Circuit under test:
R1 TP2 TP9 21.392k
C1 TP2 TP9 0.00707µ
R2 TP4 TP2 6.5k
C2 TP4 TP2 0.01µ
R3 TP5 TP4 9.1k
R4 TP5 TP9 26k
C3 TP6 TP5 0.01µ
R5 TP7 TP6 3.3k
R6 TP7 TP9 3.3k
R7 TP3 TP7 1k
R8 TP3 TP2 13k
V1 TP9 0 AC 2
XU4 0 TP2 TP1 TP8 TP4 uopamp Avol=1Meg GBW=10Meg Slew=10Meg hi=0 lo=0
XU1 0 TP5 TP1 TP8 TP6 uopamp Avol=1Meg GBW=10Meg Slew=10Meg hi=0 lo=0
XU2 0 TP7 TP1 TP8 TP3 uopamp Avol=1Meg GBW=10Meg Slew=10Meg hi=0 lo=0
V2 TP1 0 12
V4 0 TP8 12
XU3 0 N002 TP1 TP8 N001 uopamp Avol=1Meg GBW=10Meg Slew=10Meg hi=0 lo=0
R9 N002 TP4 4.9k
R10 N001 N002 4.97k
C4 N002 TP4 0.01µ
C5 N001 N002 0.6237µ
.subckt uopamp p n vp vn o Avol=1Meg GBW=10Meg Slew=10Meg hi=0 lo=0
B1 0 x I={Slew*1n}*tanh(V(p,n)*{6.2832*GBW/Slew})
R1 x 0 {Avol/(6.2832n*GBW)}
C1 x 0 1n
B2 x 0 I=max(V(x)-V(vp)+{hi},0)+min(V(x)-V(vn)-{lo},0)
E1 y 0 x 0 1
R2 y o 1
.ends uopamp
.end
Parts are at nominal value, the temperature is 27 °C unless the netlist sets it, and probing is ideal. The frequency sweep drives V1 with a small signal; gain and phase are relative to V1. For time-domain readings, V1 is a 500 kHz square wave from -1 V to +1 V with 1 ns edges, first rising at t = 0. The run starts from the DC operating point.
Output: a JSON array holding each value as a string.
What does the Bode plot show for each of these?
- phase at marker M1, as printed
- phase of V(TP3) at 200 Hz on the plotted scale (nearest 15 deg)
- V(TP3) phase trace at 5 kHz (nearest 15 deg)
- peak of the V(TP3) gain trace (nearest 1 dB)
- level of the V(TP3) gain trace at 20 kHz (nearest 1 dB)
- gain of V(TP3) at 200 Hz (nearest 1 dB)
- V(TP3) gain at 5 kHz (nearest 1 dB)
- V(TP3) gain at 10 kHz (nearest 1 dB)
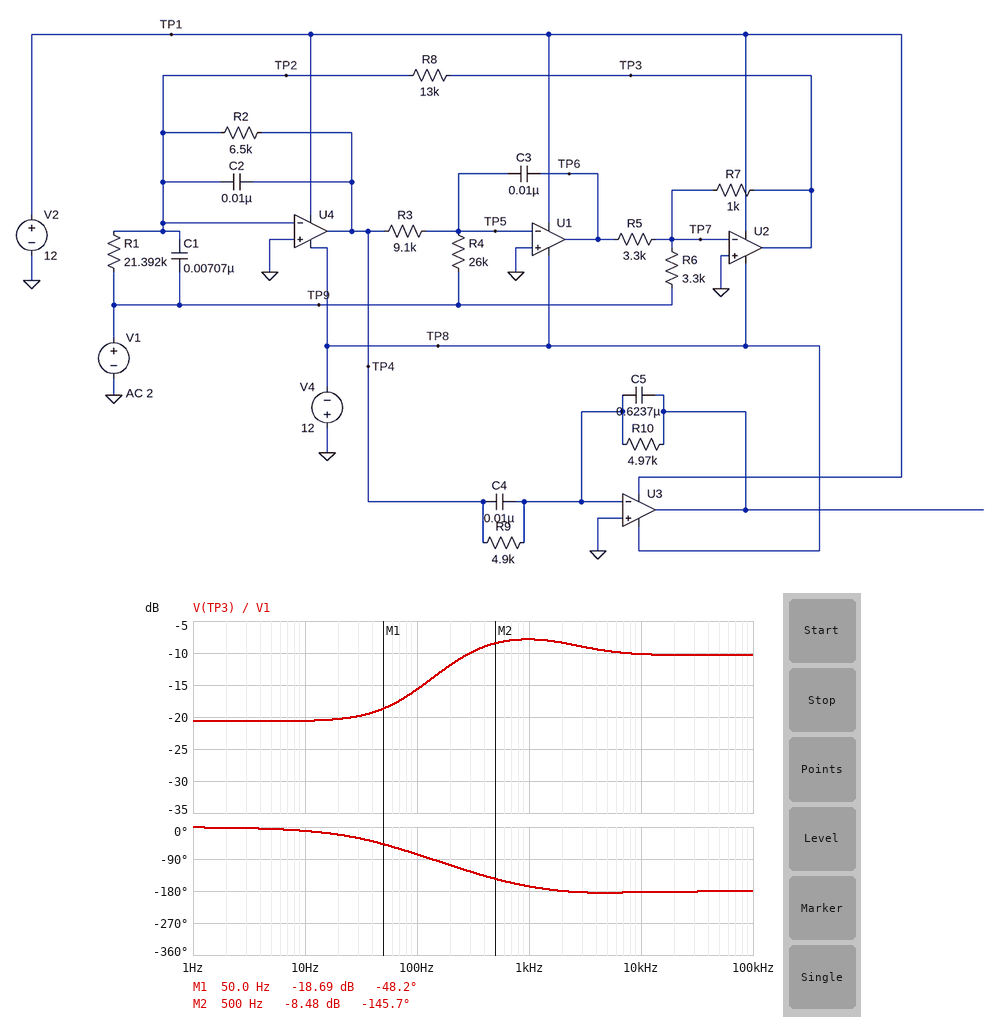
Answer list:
["-48.2 deg", "-105 deg", "-180 deg", "-8 dB", "-10 dB", "-12 dB", "-10 dB", "-10 dB"]
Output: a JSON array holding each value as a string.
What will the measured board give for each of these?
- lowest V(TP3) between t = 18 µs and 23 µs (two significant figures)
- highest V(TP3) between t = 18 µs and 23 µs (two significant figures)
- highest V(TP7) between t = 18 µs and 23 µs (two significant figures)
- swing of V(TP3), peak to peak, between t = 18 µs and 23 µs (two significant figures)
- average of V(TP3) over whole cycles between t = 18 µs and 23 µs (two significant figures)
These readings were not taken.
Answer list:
["-720 mV", "-110 mV", "370 mV", "610 mV", "-410 mV"]
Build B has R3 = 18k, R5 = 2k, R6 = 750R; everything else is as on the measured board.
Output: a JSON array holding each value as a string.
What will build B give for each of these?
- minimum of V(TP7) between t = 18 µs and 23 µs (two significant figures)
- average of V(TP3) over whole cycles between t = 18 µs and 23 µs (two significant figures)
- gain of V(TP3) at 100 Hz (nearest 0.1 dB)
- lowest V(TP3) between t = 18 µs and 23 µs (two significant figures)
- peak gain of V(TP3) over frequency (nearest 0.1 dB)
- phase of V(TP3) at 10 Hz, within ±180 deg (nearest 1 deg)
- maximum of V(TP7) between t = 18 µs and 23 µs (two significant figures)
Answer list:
["-940 mV", "-2.1 V", "-0.6 dB", "-3.4 V", "3.5 dB", "-7 deg", "940 mV"]
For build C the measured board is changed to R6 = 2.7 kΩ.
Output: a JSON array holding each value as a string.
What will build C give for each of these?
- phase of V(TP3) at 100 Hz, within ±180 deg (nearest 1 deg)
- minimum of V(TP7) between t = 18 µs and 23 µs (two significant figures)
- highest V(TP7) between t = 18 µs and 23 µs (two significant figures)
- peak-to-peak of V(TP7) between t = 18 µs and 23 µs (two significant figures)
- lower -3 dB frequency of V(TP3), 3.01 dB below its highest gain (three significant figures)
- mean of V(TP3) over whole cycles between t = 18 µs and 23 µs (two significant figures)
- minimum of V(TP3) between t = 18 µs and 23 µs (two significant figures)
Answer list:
["-81 deg", "-440 mV", "440 mV", "880 mV", "248 Hz", "-480 mV", "-850 mV"]
